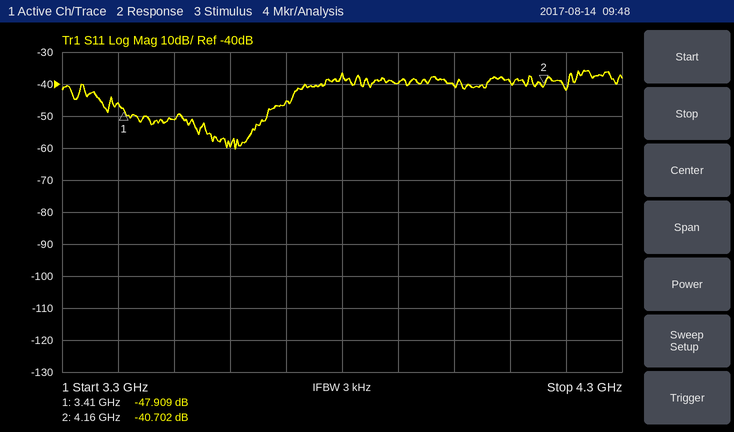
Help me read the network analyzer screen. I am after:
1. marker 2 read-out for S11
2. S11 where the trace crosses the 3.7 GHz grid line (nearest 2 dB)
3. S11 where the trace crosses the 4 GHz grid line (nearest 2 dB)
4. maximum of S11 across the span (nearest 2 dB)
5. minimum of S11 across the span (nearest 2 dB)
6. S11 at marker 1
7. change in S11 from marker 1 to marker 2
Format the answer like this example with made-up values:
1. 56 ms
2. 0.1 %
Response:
1. -40.702 dB
2. -46 dB
3. -40 dB
4. -36 dB
5. -60 dB
6. -47.909 dB
7. 7.207 dB
